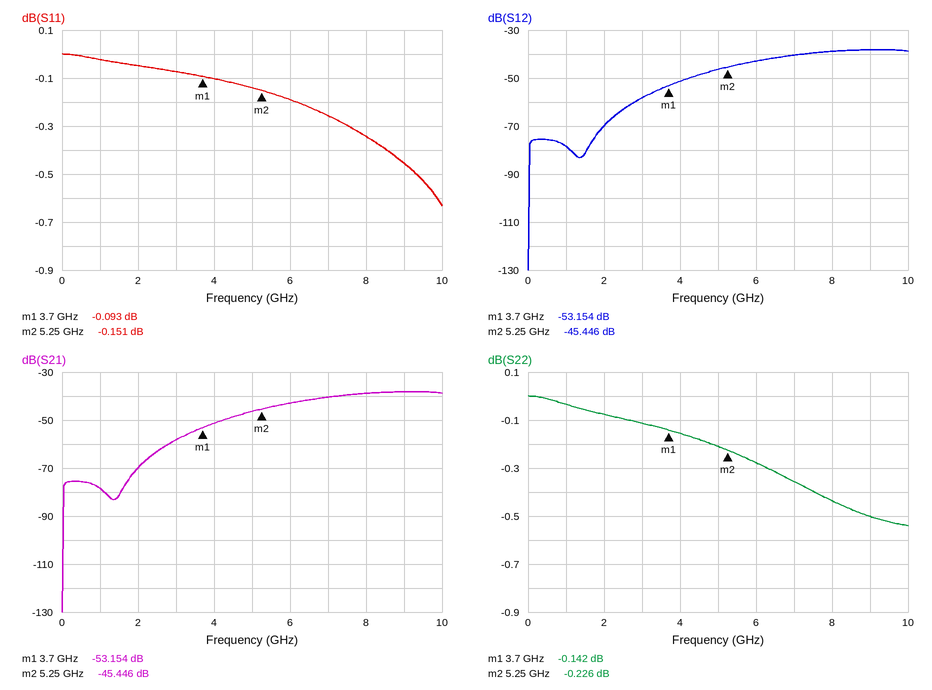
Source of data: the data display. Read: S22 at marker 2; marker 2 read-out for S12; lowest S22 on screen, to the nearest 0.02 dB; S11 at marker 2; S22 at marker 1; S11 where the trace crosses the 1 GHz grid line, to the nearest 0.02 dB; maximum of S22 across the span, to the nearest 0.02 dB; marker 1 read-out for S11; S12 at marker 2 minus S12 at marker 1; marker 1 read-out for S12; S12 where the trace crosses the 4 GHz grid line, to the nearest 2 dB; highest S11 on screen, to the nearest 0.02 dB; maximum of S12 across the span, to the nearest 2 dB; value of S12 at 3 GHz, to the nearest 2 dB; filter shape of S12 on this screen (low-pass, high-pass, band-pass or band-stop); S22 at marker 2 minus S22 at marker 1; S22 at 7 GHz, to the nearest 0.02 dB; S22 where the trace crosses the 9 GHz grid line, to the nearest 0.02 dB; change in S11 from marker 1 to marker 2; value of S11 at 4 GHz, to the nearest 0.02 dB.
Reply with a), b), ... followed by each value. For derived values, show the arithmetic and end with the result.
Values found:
a) -0.226 dB
b) -45.446 dB
c) -0.54 dB
d) -0.151 dB
e) -0.142 dB
f) -0.02 dB
g) 0.00 dB
h) -0.093 dB
i) -45.446 − (-53.154) = 7.708 dB
j) -53.154 dB
k) -52 dB
l) 0.00 dB
m) -38 dB
n) -58 dB
o) high-pass
p) -0.226 − (-0.142) = -0.084 dB
q) -0.36 dB
r) -0.50 dB
s) -0.151 − (-0.093) = -0.058 dB
t) -0.10 dB
